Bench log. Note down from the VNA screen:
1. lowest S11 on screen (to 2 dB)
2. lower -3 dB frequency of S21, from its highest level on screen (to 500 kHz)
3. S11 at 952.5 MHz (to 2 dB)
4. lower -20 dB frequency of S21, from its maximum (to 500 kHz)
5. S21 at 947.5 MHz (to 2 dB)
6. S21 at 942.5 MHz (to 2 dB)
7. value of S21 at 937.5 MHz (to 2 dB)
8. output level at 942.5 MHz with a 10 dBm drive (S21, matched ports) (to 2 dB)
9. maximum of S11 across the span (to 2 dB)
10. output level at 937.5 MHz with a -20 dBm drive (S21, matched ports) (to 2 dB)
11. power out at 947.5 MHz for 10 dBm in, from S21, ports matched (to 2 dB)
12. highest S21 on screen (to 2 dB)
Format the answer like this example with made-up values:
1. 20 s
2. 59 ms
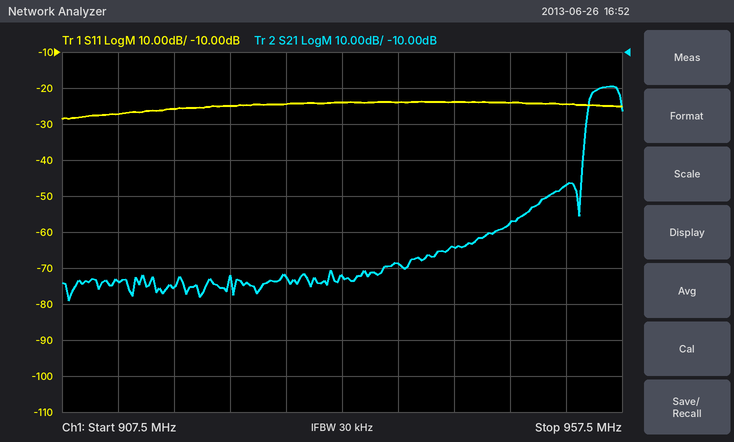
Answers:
1. -28 dB
2. 954.5 MHz
3. -24 dB
4. 954.0 MHz
5. -58 dB
6. -64 dB
7. -68 dB
8. -54 dBm
9. -24 dB
10. -88 dBm
11. -48 dBm
12. -20 dB
